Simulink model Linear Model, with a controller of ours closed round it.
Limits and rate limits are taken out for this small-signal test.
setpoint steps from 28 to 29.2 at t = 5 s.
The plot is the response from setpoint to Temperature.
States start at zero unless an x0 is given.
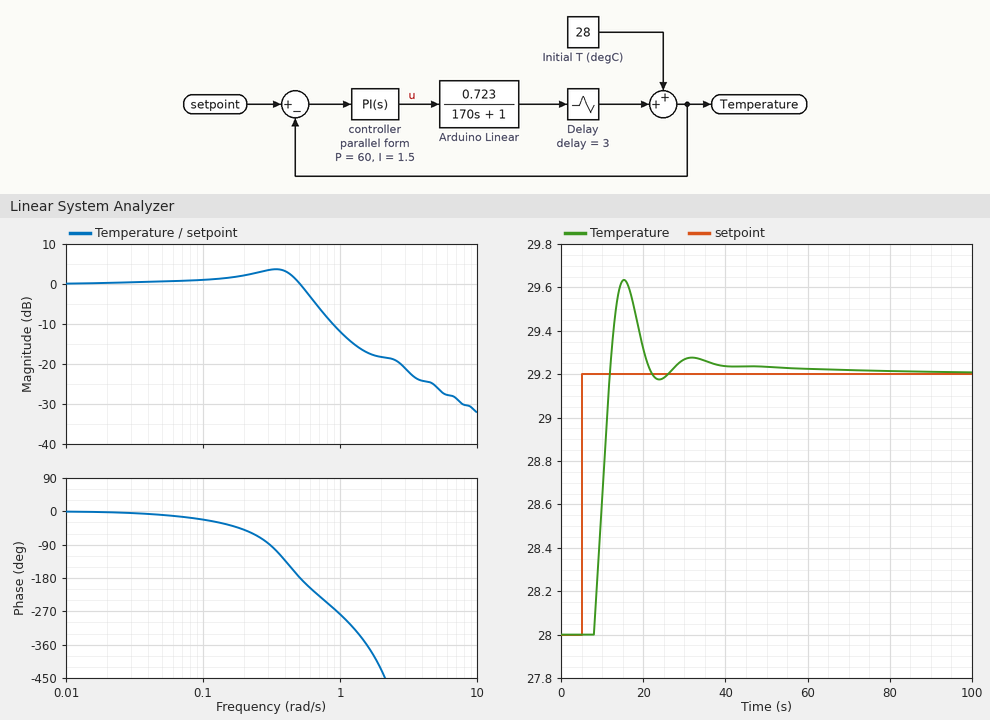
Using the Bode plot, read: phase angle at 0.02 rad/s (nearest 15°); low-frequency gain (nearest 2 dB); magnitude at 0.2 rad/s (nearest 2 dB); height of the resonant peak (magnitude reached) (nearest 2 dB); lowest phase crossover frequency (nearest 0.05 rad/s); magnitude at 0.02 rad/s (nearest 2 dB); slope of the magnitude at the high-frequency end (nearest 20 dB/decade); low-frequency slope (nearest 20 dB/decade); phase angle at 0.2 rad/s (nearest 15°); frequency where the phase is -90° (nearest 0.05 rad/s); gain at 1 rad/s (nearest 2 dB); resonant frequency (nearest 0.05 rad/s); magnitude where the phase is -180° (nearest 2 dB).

0°
0 dB
2 dB
4 dB
0.50 rad/s
0 dB
-20 dB/decade
0 dB/decade
-45°
0.30 rad/s
-12 dB
0.35 rad/s
0 dB
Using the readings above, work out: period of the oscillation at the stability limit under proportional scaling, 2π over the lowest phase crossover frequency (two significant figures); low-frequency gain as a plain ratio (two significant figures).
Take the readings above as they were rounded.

13 s
1.0
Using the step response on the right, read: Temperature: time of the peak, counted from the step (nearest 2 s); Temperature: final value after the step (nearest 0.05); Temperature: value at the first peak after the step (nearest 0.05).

10 s
29.20
29.65
